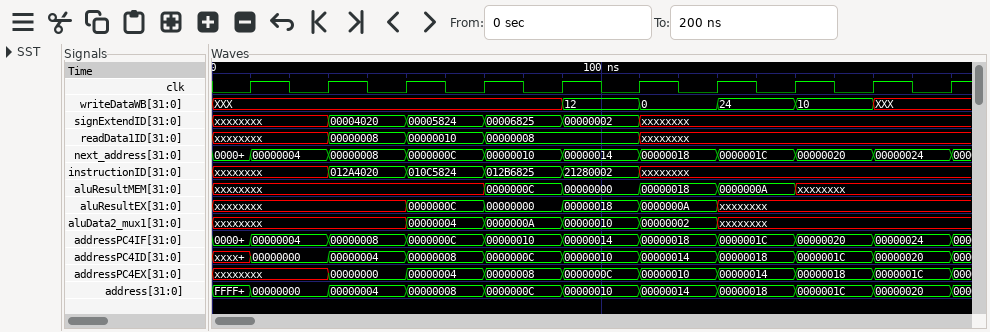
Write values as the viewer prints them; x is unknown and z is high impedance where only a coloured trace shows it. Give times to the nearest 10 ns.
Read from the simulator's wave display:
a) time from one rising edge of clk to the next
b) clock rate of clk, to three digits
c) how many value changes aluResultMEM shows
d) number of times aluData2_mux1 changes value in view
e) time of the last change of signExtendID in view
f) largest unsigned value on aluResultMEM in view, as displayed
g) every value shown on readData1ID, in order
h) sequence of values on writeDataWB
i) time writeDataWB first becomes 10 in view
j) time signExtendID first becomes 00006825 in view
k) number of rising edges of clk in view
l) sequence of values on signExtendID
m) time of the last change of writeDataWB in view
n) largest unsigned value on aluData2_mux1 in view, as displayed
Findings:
20 ns
50.0 MHz
5
5
110 ns
00000018
xxxxxxxx, 00000008, 00000010, 00000008, xxxxxxxx
XXX, 12, 0, 24, 10, XXX
150 ns
70 ns
10
xxxxxxxx, 00004020, 00005824, 00006825, 00000002, xxxxxxxx
170 ns
00000010
